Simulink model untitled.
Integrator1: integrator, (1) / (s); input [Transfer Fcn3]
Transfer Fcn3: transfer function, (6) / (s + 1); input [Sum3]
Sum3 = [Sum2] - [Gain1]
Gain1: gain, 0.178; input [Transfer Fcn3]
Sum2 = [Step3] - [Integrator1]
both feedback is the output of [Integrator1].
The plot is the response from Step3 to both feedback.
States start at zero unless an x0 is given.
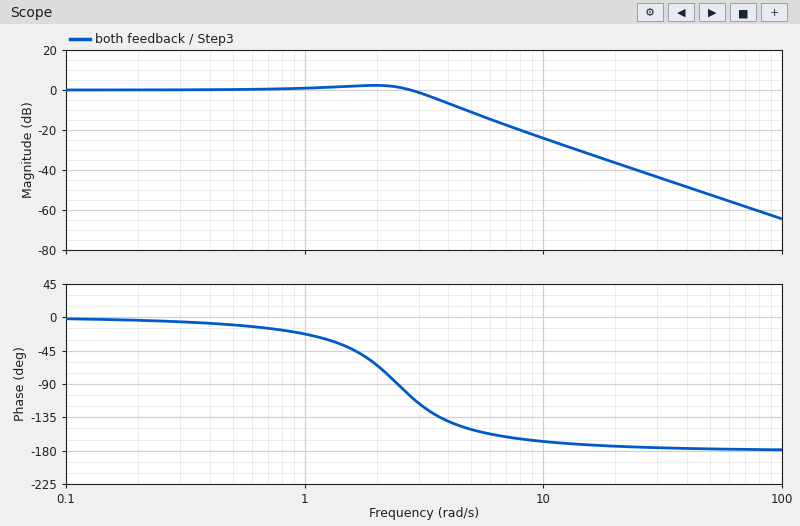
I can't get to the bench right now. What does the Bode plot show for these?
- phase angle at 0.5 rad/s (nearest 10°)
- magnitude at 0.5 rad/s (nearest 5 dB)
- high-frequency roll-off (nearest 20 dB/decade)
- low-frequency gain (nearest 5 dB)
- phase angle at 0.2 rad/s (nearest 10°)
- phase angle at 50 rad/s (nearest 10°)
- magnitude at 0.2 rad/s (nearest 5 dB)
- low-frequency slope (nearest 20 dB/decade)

-10°
0 dB
-40 dB/decade
0 dB
0°
-180°
0 dB
0 dB/decade
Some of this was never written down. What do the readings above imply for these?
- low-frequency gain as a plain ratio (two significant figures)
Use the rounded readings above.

1.0
